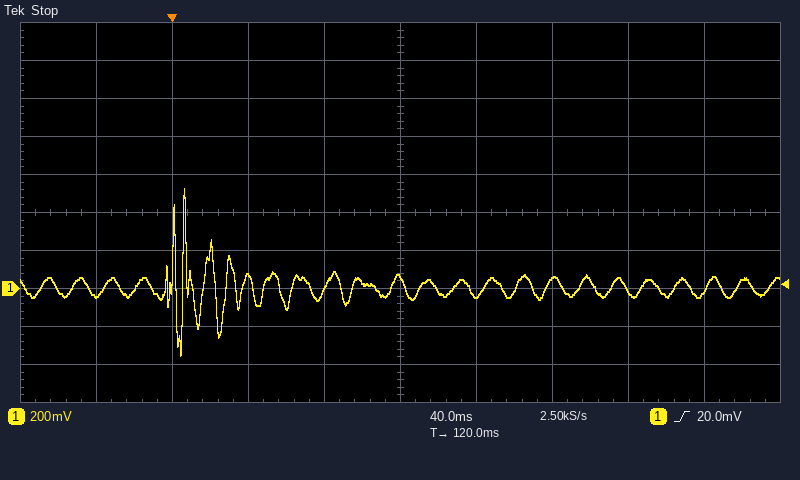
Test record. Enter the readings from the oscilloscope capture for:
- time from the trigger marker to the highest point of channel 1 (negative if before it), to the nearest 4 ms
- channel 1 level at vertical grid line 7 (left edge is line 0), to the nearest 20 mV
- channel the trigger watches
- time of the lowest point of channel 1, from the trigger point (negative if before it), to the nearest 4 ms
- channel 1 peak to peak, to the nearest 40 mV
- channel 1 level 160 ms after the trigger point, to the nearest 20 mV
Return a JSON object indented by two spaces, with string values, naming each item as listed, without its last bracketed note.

{
  "time from the trigger marker to the highest point of channel 1 (negative if before it), to the nearest 4 ms": "+8 ms",
  "channel 1 level at vertical grid line 7 (left edge is line 0), to the nearest 20 mV": "40 mV",
  "channel the trigger watches": "channel 1",
  "time of the lowest point of channel 1, from the trigger point (negative if before it), to the nearest 4 ms": "+4 ms",
  "channel 1 peak to peak, to the nearest 40 mV": "880 mV",
  "channel 1 level 160 ms after the trigger point, to the nearest 20 mV": "-40 mV"
}
